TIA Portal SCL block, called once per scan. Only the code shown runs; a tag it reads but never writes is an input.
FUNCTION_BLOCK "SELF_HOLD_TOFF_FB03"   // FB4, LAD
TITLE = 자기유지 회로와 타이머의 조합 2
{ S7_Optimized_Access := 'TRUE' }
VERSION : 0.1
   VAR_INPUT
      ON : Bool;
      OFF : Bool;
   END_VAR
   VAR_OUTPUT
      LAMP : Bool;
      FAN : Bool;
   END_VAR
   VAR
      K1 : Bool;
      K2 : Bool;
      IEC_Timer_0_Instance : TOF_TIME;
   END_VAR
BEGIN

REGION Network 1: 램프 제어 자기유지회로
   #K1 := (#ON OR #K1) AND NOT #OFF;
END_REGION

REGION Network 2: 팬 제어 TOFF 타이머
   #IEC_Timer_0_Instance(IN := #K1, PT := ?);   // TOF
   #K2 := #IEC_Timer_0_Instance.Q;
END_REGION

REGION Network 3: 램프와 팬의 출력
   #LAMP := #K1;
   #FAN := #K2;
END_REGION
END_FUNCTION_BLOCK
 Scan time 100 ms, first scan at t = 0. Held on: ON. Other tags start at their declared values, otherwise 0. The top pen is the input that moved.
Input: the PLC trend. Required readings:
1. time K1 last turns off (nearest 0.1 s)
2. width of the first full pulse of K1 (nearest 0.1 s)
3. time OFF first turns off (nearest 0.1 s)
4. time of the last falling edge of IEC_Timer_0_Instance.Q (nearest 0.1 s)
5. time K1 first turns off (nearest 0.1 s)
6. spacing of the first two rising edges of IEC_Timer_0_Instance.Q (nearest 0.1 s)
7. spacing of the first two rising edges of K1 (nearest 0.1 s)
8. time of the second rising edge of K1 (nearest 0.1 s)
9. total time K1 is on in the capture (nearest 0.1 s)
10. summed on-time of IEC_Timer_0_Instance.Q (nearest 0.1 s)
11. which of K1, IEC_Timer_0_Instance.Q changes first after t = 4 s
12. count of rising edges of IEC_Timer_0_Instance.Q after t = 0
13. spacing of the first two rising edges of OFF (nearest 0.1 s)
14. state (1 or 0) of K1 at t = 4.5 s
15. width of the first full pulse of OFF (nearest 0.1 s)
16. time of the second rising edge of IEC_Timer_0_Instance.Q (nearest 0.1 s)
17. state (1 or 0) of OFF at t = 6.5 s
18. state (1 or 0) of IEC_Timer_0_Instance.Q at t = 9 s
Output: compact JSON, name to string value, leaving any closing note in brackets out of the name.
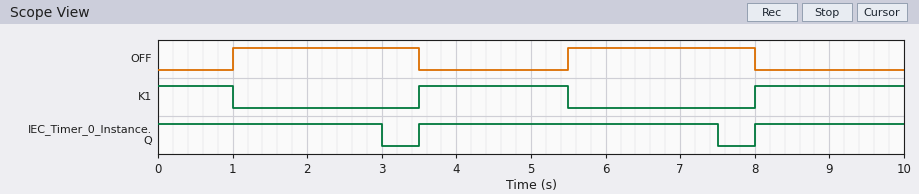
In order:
{"time K1 last turns off": "5.5 s", "width of the first full pulse of K1": "2.0 s", "time OFF first turns off": "3.5 s", "time of the last falling edge of IEC_Timer_0_Instance.Q": "7.5 s", "time K1 first turns off": "1.0 s", "spacing of the first two rising edges of IEC_Timer_0_Instance.Q": "4.5 s", "spacing of the first two rising edges of K1": "4.5 s", "time of the second rising edge of K1": "8.0 s", "total time K1 is on in the capture": "5.0 s", "summed on-time of IEC_Timer_0_Instance.Q": "9.0 s", "which of K1, IEC_Timer_0_Instance.Q changes first after t = 4 s": "K1", "count of rising edges of IEC_Timer_0_Instance.Q after t = 0": "2", "spacing of the first two rising edges of OFF": "4.5 s", "state (1 or 0) of K1 at t = 4.5 s": "1", "width of the first full pulse of OFF": "2.5 s", "time of the second rising edge of IEC_Timer_0_Instance.Q": "8.0 s", "state (1 or 0) of OFF at t = 6.5 s": "1", "state (1 or 0) of IEC_Timer_0_Instance.Q at t = 9 s": "1"}
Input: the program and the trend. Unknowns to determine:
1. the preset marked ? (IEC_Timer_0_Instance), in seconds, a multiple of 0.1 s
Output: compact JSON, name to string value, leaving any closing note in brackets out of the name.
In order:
{"the preset marked ? (IEC_Timer_0_Instance), in seconds, a multiple of 0.1 s": "2.0 s"}
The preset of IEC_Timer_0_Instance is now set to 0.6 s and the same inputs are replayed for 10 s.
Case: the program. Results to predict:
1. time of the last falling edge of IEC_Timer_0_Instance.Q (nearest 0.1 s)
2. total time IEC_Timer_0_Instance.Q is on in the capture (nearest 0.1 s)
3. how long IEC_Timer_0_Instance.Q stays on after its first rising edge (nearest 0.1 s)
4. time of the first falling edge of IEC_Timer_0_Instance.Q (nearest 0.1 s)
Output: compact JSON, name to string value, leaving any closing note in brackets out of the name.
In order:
{"time of the last falling edge of IEC_Timer_0_Instance.Q": "6.1 s", "total time IEC_Timer_0_Instance.Q is on in the capture": "6.2 s", "how long IEC_Timer_0_Instance.Q stays on after its first rising edge": "2.6 s", "time of the first falling edge of IEC_Timer_0_Instance.Q": "1.6 s"}
